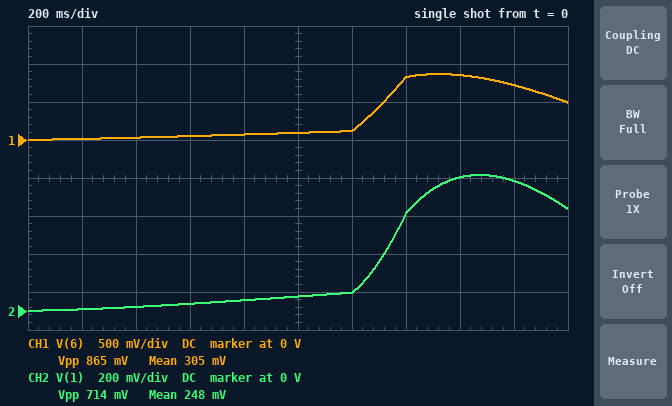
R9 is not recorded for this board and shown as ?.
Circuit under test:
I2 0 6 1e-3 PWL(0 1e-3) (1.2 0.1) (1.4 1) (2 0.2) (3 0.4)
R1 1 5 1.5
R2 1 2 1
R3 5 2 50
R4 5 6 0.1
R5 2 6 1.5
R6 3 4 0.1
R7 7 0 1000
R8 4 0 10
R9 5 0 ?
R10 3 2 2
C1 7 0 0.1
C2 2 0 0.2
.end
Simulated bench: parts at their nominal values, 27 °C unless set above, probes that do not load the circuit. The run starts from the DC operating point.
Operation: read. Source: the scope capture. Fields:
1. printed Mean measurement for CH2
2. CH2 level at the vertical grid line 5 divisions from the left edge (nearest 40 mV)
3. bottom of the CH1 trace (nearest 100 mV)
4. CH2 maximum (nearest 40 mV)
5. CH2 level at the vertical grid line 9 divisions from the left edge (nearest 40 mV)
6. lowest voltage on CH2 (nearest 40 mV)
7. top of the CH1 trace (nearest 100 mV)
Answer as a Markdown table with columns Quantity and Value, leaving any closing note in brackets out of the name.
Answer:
| Quantity | Value |
|---|---|
| printed Mean measurement for CH2 | 248 mV |
| CH2 level at the vertical grid line 5 divisions from the left edge | 80 mV |
| bottom of the CH1 trace | 0 V |
| CH2 maximum | 720 mV |
| CH2 level at the vertical grid line 9 divisions from the left edge | 680 mV |
| lowest voltage on CH2 | 0 V |
| top of the CH1 trace | 900 mV |
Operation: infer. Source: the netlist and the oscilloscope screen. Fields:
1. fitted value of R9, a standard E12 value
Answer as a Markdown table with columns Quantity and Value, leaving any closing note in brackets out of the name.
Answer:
| Quantity | Value |
|---|---|
| fitted value of R9, a standard E12 value | 1.5 Ω |
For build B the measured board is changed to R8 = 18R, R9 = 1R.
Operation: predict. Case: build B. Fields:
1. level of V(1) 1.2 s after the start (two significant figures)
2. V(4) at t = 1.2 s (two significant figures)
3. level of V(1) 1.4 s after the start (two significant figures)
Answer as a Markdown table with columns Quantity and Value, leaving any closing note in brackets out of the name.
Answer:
| Quantity | Value |
|---|---|
| level of V(1) 1.2 s after the start | 74 mV |
| V(4) at t = 1.2 s | 62 mV |
| level of V(1) 1.4 s after the start | 410 mV |
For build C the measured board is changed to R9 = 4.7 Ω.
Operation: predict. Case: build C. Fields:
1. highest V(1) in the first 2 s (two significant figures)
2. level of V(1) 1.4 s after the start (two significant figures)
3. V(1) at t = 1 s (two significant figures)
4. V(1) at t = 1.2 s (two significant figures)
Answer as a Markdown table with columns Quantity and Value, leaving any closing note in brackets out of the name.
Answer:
| Quantity | Value |
|---|---|
| highest V(1) in the first 2 s | 1.3 V |
| level of V(1) 1.4 s after the start | 810 mV |
| V(1) at t = 1 s | 140 mV |
| V(1) at t = 1.2 s | 180 mV |
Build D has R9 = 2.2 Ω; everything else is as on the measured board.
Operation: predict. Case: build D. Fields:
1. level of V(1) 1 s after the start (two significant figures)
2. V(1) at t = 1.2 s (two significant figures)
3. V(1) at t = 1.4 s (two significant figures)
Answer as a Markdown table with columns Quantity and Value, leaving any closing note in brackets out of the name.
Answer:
| Quantity | Value |
|---|---|
| level of V(1) 1 s after the start | 96 mV |
| V(1) at t = 1.2 s | 120 mV |
| V(1) at t = 1.4 s | 620 mV |
